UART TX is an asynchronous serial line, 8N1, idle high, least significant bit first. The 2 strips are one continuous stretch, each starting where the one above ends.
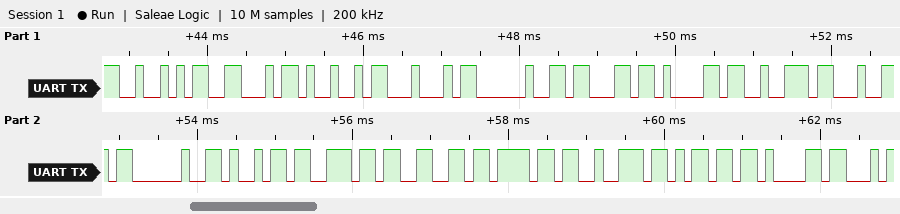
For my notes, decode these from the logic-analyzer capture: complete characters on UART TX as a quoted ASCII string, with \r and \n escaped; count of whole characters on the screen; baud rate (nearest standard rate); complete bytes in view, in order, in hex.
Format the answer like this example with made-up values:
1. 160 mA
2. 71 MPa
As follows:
1. "RFID card informa"
2. 17
3. 9600 baud
4. 52 46 49 44 20 63 61 72 64 20 69 6E 66 6F 72 6D 61
